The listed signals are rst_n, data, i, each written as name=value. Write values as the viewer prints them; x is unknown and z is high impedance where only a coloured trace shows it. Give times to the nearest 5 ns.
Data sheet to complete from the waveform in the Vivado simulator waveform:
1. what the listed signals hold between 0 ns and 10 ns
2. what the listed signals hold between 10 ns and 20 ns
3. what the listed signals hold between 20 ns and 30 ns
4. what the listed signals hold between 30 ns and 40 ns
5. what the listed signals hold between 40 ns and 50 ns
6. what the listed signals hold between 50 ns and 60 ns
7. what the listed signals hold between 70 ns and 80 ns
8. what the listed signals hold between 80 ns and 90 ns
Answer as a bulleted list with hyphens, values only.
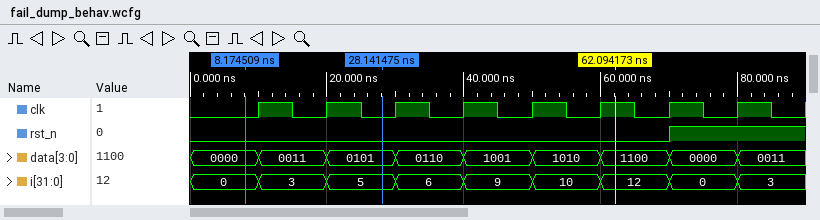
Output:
- rst_n=0, data=0000, i=0
- rst_n=0, data=0011, i=3
- rst_n=0, data=0101, i=5
- rst_n=0, data=0110, i=6
- rst_n=0, data=1001, i=9
- rst_n=0, data=1010, i=10
- rst_n=1, data=0000, i=0
- rst_n=1, data=0011, i=3
